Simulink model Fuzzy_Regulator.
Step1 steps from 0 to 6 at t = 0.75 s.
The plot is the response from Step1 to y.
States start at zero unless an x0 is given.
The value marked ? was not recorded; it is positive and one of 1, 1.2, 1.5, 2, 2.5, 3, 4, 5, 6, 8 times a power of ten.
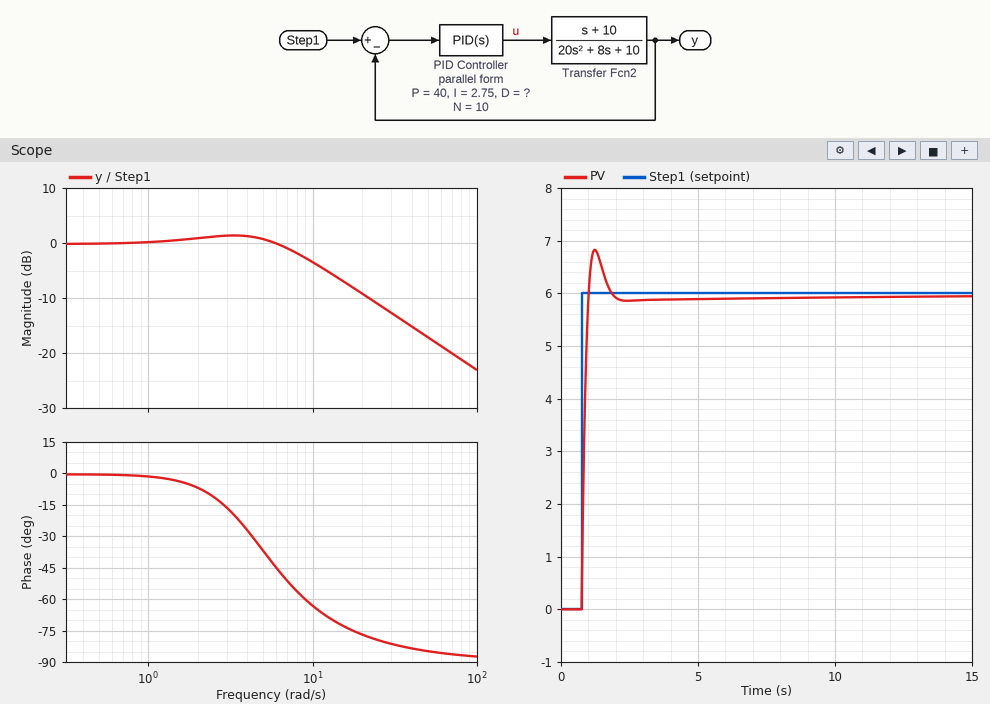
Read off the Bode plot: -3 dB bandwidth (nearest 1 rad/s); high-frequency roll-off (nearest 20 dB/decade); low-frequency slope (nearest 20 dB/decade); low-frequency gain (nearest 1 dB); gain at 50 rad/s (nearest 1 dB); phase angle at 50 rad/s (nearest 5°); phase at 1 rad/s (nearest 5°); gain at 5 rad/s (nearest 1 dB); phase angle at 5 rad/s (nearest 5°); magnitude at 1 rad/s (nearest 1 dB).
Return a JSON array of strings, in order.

["10 rad/s", "-20 dB/decade", "0 dB/decade", "0 dB", "-17 dB", "-85°", "0°", "1 dB", "-35°", "0 dB"]
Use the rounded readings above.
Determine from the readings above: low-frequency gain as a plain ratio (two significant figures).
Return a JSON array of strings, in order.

["1.0"]
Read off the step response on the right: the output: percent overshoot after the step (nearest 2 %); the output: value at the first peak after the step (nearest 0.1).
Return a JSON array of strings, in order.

["14 %", "6.8"]
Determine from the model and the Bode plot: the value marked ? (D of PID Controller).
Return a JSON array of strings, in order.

["10"]
